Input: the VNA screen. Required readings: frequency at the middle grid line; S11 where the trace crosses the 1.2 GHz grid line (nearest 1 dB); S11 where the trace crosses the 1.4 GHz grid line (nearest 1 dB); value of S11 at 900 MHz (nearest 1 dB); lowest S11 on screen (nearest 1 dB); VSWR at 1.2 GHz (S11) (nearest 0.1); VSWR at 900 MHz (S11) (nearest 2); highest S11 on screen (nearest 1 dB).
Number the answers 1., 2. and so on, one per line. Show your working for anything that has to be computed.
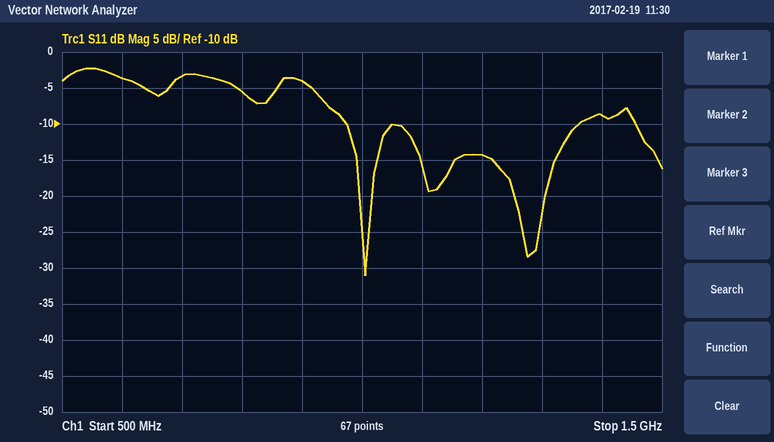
1. 1 GHz
2. -14 dB
3. -9 dB
4. -4 dB
5. -31 dB
6. |Γ| = 10^(-14/20) = 0.1995; VSWR = (1 + 0.1995)/(1 − 0.1995) ≈ 1.5
7. |Γ| = 10^(-4/20) = 0.6310; VSWR = (1 + 0.6310)/(1 − 0.6310) ≈ 4
8. -2 dB
